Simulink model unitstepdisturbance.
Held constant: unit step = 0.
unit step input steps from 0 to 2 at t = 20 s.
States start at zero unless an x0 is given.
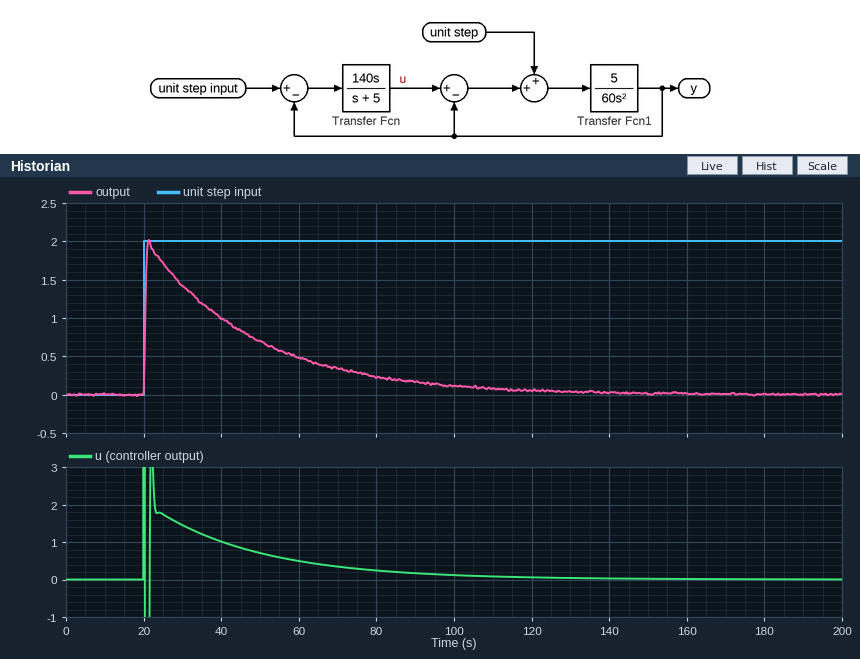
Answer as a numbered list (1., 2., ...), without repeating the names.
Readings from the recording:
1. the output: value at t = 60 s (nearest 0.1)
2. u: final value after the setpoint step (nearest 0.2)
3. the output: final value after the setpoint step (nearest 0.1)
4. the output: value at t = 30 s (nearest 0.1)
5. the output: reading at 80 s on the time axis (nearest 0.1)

1. 0.5
2. 0.0
3. 0.0
4. 1.4
5. 0.2
